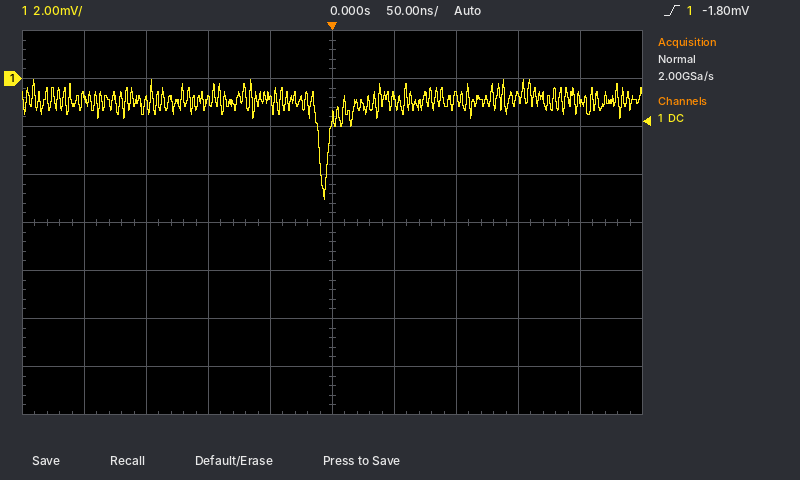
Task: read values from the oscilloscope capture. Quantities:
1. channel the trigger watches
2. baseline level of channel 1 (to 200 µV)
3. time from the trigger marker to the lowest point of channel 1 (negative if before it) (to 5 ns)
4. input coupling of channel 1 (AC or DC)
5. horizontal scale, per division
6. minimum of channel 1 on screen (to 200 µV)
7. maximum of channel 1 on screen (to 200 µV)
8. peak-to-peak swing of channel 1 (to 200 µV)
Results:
channel 1
-1.0 mV
-5 ns
DC
50 ns
-5.0 mV
0.0 mV
5.0 mV
